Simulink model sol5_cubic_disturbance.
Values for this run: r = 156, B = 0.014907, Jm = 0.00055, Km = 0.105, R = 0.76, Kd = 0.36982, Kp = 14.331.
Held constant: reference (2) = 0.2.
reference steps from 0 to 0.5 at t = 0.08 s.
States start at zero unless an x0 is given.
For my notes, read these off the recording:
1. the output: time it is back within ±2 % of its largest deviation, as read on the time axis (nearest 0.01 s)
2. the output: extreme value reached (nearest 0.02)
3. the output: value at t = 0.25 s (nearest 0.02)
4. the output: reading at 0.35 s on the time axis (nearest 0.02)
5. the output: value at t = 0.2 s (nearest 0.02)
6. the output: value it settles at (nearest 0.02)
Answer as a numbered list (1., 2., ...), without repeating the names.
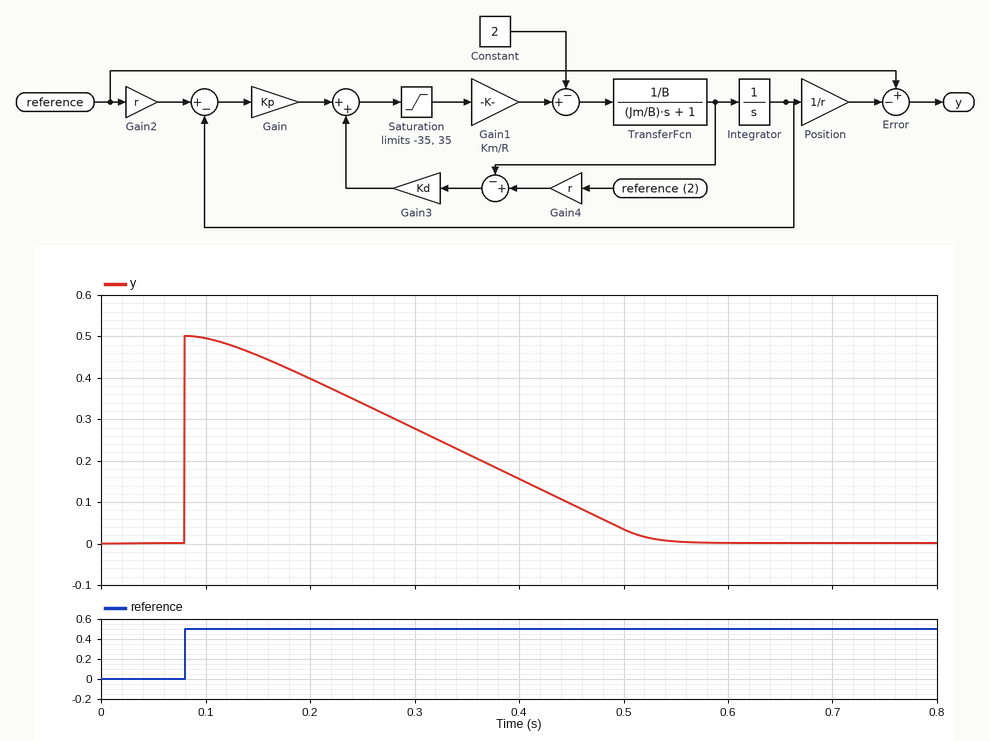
1. 0.53 s
2. 0.50
3. 0.34
4. 0.22
5. 0.40
6. 0.00
